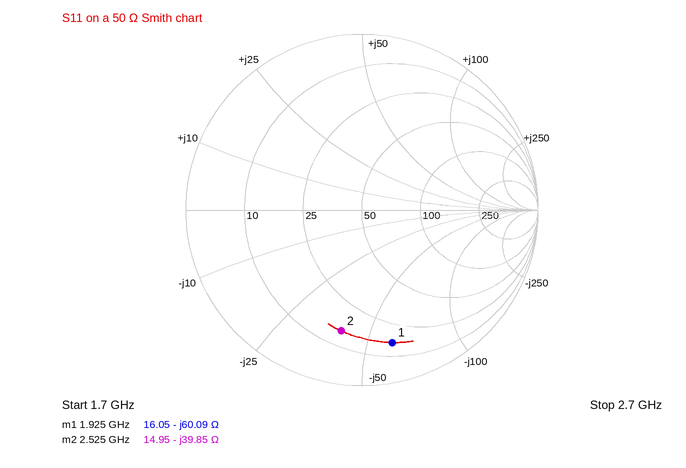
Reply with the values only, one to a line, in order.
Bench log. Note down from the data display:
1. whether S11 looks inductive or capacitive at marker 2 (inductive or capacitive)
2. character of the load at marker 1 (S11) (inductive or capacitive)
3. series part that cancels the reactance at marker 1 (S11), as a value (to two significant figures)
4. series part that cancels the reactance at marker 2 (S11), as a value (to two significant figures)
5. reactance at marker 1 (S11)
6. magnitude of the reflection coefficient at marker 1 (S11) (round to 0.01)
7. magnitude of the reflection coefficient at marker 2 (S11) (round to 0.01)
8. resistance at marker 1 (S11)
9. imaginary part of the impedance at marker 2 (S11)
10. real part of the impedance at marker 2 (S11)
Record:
capacitive
capacitive
5.0 nH
2.5 nH
-60.09 Ω
0.77
0.70
16.05 Ω
-39.85 Ω
14.95 Ω
